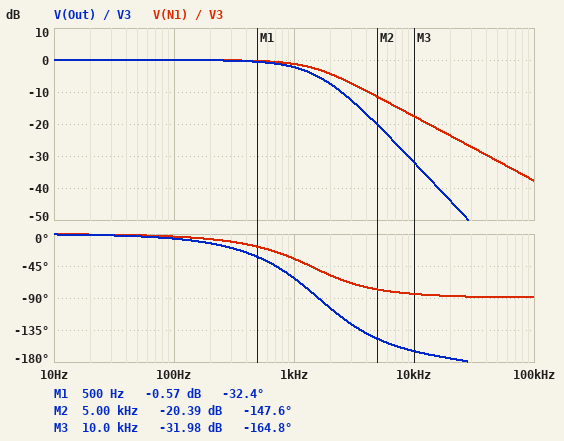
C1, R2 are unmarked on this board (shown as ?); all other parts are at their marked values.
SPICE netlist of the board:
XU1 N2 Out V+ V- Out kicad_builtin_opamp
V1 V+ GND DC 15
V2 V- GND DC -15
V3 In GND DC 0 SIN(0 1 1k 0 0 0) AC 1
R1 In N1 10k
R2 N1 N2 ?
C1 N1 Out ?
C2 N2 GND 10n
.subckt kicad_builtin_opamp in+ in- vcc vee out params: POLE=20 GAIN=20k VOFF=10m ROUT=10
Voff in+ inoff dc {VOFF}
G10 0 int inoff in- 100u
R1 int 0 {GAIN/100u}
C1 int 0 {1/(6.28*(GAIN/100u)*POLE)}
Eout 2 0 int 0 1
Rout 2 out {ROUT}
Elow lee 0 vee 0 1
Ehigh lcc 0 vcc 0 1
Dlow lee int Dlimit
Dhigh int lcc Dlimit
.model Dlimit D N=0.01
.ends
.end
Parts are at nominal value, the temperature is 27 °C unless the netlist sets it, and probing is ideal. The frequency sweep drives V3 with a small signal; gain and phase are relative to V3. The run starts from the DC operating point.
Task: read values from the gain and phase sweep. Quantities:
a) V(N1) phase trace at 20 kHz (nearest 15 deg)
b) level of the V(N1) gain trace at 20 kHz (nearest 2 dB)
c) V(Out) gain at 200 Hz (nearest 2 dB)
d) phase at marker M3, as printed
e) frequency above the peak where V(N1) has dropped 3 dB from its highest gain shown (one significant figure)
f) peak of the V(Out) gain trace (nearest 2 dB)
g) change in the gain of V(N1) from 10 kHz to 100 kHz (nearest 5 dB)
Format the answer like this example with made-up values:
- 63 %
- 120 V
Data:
- -90 deg
- -24 dB
- 0 dB
- -164.8 deg
- 2 kHz
- 0 dB
- -20 dB
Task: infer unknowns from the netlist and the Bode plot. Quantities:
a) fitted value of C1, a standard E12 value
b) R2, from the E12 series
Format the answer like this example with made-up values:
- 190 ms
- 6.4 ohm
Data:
- 12 nF
- 8.2 kΩ
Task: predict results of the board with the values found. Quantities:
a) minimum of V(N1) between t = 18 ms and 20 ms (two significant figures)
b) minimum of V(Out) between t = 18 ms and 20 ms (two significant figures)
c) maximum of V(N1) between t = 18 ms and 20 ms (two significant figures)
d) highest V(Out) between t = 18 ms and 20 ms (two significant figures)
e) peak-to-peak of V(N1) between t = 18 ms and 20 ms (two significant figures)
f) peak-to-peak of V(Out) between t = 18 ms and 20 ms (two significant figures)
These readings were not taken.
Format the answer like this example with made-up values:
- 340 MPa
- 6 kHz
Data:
- -870 mV
- -780 mV
- 870 mV
- 760 mV
- 1.7 V
- 1.5 V
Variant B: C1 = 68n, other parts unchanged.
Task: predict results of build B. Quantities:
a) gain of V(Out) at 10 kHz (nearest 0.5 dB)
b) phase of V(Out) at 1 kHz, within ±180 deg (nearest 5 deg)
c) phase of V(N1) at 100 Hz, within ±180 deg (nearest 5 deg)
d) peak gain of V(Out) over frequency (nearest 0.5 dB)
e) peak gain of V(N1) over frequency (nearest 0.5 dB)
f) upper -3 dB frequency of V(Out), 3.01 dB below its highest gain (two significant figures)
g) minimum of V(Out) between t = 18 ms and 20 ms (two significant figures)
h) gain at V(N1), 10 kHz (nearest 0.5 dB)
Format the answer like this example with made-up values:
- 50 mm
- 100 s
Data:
- -47.0 dB
- -135 deg
- -5 deg
- 3.0 dB
- 3.5 dB
- 800 Hz
- -610 mV
- -32.5 dB
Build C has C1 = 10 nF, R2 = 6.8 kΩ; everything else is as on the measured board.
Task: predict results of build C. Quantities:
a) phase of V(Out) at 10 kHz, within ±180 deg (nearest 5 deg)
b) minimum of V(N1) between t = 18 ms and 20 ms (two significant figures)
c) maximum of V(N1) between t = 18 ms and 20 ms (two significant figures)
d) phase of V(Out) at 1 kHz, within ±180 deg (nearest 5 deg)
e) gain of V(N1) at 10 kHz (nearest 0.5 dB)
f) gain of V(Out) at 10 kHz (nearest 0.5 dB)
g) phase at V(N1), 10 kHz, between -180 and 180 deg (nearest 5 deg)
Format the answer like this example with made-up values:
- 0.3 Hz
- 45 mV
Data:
- -160 deg
- -850 mV
- 850 mV
- -55 deg
- -16.0 dB
- -29.0 dB
- -80 deg
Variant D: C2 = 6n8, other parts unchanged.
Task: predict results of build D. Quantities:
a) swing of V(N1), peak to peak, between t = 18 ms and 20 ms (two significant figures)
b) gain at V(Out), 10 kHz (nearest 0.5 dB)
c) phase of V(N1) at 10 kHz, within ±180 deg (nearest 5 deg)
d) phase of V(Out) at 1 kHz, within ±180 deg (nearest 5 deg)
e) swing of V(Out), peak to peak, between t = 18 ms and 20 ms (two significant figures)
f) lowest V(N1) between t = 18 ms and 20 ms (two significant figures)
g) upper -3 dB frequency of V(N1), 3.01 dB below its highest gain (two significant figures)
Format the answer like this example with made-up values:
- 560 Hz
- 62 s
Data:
- 2.0 V
- -28.5 dB
- -90 deg
- -45 deg
- 1.9 V
- -990 mV
- 2.3 kHz
